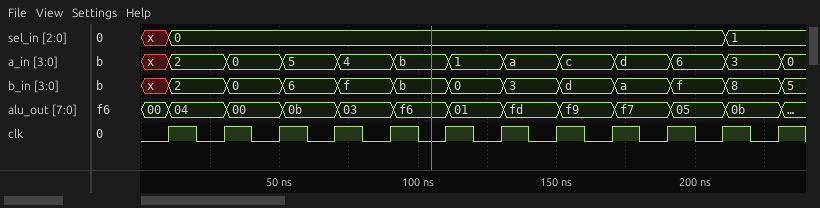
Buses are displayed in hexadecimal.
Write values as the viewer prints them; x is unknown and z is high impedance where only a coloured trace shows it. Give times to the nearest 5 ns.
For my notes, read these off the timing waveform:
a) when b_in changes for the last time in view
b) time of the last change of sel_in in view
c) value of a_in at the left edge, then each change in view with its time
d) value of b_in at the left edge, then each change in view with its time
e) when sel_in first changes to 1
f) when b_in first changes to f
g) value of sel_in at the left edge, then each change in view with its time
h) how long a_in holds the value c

230 ns
210 ns
x, 2 at 10 ns, 0 at 30 ns, 5 at 50 ns, 4 at 70 ns, b at 90 ns, 1 at 110 ns, a at 130 ns, c at 150 ns, d at 170 ns, 6 at 190 ns, 3 at 210 ns, 0 at 230 ns
x, 2 at 10 ns, 0 at 30 ns, 6 at 50 ns, f at 70 ns, b at 90 ns, 0 at 110 ns, 3 at 130 ns, d at 150 ns, a at 170 ns, f at 190 ns, 8 at 210 ns, 5 at 230 ns
210 ns
70 ns
x, 0 at 10 ns, 1 at 210 ns
20 ns
